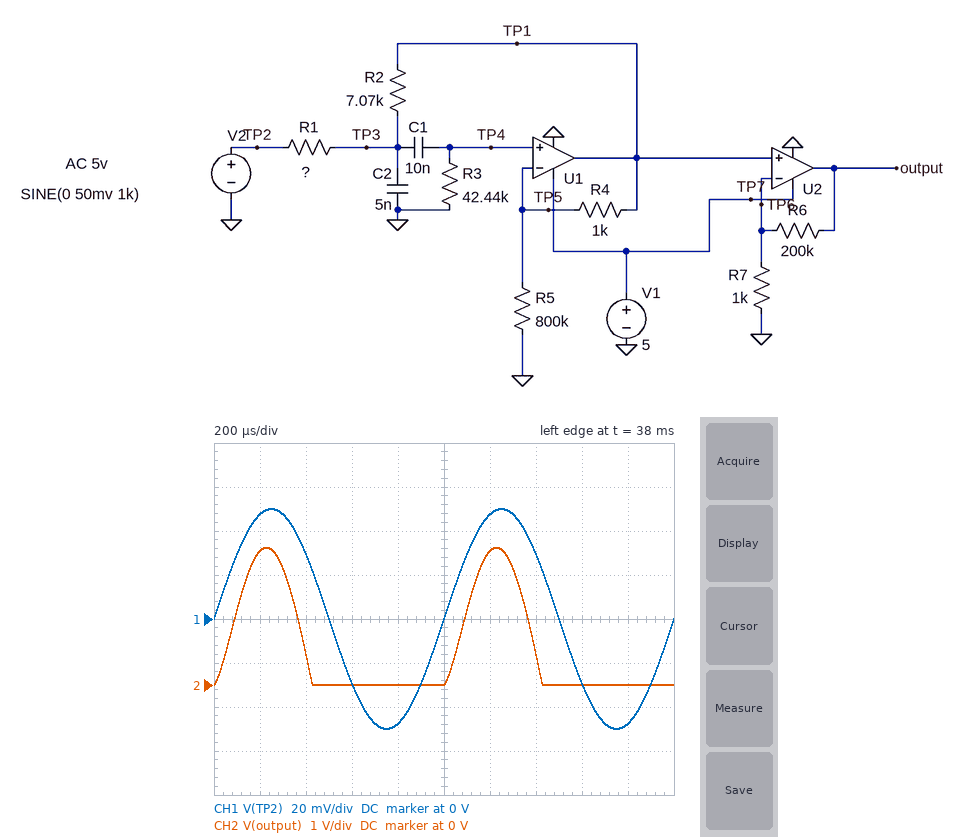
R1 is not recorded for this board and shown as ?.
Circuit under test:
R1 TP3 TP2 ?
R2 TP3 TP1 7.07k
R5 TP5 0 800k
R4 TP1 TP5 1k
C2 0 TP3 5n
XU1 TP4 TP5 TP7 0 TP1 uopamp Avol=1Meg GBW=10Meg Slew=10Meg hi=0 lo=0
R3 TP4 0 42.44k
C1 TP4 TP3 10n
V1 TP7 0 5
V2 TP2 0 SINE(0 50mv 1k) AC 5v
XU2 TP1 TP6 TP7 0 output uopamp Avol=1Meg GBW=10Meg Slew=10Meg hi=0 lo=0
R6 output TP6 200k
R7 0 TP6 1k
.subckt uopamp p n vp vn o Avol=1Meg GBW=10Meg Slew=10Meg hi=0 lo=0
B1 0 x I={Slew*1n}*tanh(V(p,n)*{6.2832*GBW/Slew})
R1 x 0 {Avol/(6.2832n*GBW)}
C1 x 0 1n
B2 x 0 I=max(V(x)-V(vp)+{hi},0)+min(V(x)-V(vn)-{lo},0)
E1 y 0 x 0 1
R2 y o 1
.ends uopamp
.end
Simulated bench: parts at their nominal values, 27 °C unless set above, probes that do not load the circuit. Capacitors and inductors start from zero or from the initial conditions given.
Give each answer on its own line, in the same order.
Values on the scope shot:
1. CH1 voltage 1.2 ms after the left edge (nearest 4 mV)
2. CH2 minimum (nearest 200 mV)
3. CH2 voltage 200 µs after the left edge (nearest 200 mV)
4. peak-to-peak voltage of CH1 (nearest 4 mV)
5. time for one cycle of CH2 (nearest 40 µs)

48 mV
0 V
3.0 V
100 mV
1.00 ms
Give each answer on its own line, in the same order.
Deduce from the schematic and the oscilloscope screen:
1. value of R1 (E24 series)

30 kΩ
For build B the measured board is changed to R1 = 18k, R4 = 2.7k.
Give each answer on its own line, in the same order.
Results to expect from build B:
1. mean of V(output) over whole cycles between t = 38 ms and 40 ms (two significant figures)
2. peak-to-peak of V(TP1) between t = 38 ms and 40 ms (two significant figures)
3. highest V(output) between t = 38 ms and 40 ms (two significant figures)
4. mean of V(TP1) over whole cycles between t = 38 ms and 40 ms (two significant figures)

1.1 V
22 mV
4.3 V
5.3 mV
